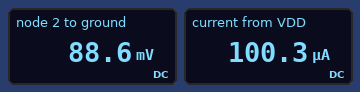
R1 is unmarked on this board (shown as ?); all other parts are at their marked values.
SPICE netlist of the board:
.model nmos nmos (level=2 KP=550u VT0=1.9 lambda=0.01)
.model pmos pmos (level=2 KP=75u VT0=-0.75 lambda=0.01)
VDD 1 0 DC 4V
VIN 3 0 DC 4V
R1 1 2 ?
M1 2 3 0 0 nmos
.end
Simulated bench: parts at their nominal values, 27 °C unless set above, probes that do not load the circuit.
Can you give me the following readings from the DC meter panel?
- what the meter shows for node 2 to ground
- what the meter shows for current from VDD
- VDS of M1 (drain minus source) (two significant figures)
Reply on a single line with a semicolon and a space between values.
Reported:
88.6 mV; 100.3 µA; 89 mV
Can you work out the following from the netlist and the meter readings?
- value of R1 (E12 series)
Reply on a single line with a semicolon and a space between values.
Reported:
39 kΩ
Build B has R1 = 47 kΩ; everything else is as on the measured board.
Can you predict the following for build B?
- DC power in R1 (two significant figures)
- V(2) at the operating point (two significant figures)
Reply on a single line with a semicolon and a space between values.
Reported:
330 µW; 74 mV
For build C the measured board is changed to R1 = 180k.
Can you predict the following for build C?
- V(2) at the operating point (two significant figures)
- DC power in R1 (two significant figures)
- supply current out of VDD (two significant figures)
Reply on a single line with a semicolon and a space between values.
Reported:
19 mV; 88 µW; 22 µA
